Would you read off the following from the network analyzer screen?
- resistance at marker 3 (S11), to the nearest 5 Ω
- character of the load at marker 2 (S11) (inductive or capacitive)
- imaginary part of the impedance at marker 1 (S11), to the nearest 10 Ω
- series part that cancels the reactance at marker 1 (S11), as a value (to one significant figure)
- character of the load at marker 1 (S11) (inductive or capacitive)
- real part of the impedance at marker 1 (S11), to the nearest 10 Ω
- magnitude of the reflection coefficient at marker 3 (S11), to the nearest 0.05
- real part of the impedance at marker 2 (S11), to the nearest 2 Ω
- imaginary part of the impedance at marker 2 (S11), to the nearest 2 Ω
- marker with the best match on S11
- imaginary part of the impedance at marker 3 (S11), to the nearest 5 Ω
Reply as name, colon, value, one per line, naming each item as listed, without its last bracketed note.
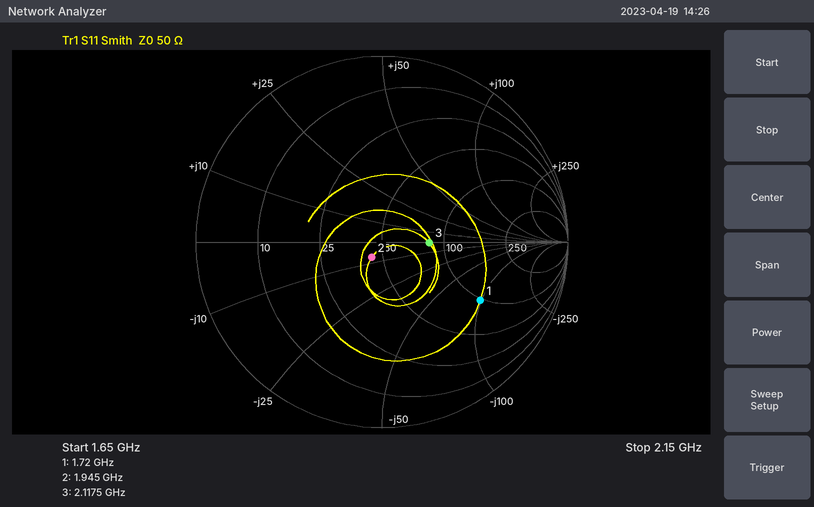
resistance at marker 3 (S11), to the nearest 5 Ω: 85 Ω
character of the load at marker 2 (S11): capacitive
imaginary part of the impedance at marker 1 (S11), to the nearest 10 Ω: -100 Ω
series part that cancels the reactance at marker 1 (S11), as a value: 9 nH
character of the load at marker 1 (S11): capacitive
real part of the impedance at marker 1 (S11), to the nearest 10 Ω: 100 Ω
magnitude of the reflection coefficient at marker 3 (S11), to the nearest 0.05: 0.25
real part of the impedance at marker 2 (S11), to the nearest 2 Ω: 44 Ω
imaginary part of the impedance at marker 2 (S11), to the nearest 2 Ω: -8 Ω
marker with the best match on S11: marker 2
imaginary part of the impedance at marker 3 (S11), to the nearest 5 Ω: 0 Ω
